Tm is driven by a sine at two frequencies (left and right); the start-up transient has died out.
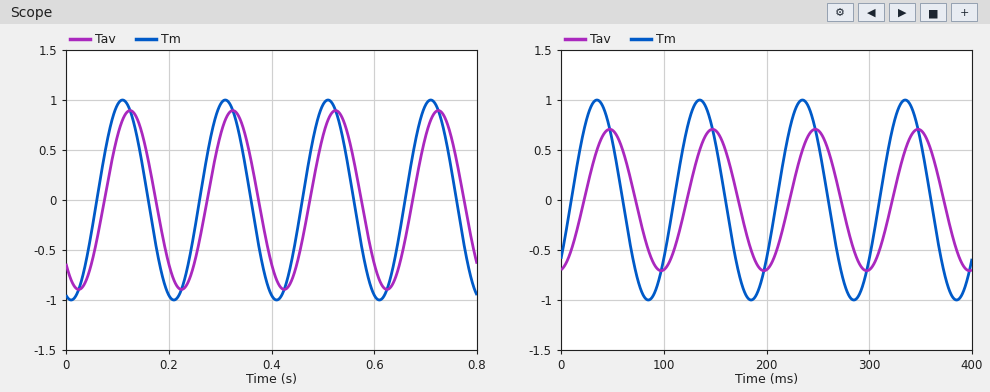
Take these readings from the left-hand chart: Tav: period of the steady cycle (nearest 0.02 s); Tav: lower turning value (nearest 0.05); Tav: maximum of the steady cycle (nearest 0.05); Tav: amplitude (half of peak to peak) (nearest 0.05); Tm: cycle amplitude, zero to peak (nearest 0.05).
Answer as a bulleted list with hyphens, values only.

- 0.20 s
- -0.90
- 0.90
- 0.90
- 1.00
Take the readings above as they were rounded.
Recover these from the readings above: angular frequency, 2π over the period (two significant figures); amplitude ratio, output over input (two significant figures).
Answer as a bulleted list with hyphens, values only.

- 31 rad/s
- 0.90
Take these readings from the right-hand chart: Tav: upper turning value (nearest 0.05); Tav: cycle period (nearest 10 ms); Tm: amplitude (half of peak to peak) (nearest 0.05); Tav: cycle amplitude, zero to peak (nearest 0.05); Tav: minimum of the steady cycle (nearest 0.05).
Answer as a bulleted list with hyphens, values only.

- 0.70
- 100 ms
- 1.00
- 0.70
- -0.70
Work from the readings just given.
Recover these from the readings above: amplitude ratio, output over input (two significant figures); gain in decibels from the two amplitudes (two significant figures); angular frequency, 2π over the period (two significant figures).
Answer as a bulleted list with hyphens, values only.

- 0.70
- -3.1 dB
- 0.063 rad/ms
